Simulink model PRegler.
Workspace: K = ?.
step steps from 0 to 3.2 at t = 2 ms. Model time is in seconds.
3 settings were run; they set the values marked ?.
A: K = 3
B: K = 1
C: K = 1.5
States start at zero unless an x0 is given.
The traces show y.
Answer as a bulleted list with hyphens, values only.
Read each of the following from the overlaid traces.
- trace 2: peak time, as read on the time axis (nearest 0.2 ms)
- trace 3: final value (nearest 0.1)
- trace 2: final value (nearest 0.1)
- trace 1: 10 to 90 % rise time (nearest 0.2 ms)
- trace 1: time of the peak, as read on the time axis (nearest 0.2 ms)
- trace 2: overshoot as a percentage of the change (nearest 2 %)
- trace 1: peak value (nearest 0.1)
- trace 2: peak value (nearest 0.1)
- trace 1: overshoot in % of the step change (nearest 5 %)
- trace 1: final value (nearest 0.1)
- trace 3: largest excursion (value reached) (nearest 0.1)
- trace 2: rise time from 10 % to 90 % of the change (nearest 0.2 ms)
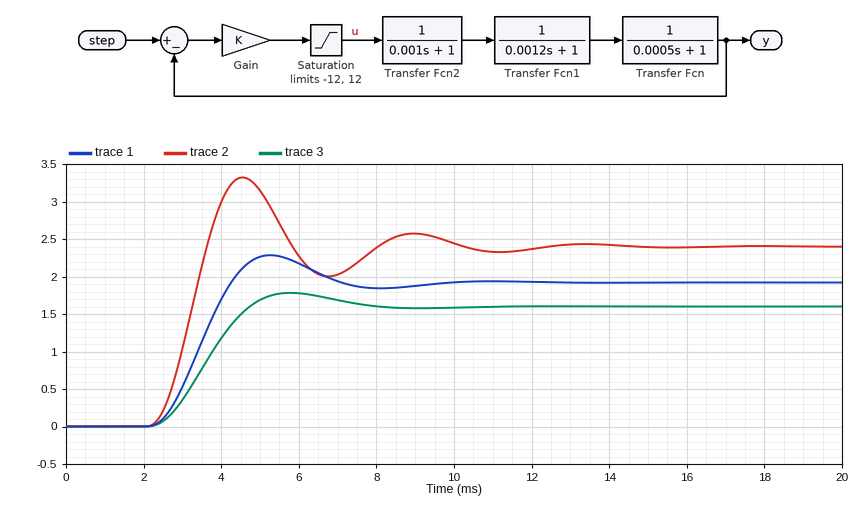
- 4.6 ms
- 1.6
- 2.4
- 1.4 ms
- 5.2 ms
- 38 %
- 2.3
- 3.3
- 20 %
- 1.9
- 1.8
- 1.0 ms
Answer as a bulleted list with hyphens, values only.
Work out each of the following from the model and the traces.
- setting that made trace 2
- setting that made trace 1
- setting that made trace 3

- A
- C
- B
